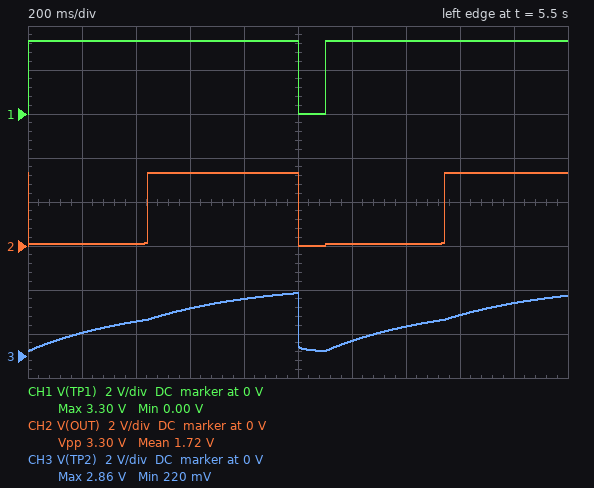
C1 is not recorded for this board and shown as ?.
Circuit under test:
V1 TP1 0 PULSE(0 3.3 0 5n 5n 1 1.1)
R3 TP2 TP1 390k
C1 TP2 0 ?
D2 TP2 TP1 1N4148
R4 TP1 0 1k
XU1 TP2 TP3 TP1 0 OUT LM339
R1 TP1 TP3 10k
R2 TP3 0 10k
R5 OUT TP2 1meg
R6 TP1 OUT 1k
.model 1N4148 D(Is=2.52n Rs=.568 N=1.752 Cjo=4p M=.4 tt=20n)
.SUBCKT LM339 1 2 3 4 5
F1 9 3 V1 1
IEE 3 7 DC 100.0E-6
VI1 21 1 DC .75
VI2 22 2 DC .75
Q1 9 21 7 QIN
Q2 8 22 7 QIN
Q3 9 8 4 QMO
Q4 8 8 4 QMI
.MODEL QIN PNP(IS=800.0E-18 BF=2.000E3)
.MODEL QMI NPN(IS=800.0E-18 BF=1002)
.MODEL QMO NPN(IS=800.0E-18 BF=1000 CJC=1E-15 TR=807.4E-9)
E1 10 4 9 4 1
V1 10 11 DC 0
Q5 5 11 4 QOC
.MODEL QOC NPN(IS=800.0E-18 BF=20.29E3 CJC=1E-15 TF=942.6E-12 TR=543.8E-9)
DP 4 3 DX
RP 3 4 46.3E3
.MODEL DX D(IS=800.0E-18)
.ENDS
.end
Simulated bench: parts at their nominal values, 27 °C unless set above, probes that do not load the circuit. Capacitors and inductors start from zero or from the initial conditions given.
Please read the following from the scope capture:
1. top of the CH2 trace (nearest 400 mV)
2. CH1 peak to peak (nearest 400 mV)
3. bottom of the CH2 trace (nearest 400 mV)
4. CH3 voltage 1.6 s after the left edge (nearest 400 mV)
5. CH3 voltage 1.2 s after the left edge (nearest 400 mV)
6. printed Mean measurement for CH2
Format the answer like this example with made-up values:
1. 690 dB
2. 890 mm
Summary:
1. 3.2 V
2. 3.2 V
3. 0 V
4. 2.0 V
5. 800 mV
6. 1.72 V
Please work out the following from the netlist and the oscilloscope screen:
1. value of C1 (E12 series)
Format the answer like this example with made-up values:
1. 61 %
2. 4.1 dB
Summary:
1. 1.5 µF
